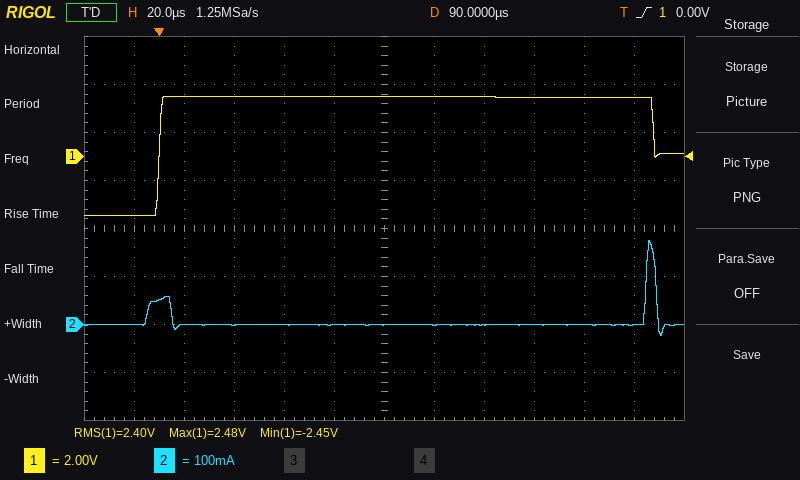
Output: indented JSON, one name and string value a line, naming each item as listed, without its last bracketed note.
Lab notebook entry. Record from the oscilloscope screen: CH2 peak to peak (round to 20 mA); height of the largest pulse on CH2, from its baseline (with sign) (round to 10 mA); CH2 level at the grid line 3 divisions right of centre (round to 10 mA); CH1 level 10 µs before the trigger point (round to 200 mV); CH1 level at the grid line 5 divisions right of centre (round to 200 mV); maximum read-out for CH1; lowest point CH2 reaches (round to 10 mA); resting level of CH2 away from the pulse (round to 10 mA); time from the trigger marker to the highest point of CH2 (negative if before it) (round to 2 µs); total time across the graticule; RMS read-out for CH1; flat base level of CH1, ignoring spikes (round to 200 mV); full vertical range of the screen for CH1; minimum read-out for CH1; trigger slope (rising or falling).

{
  "CH2 peak to peak": "200 mA",
  "height of the largest pulse on CH2, from its baseline (with sign)": "+180 mA",
  "CH2 level at the grid line 3 divisions right of centre": "0 mA",
  "CH1 level 10 µs before the trigger point": "-2.4 V",
  "CH1 level at the grid line 5 divisions right of centre": "2.4 V",
  "maximum read-out for CH1": "2.48 V",
  "lowest point CH2 reaches": "-20 mA",
  "resting level of CH2 away from the pulse": "0 mA",
  "time from the trigger marker to the highest point of CH2 (negative if before it)": "+196 µs",
  "total time across the graticule": "240 µs",
  "RMS read-out for CH1": "2.40 V",
  "flat base level of CH1, ignoring spikes": "-2.4 V",
  "full vertical range of the screen for CH1": "16 V",
  "minimum read-out for CH1": "-2.45 V",
  "trigger slope": "rising"
}
